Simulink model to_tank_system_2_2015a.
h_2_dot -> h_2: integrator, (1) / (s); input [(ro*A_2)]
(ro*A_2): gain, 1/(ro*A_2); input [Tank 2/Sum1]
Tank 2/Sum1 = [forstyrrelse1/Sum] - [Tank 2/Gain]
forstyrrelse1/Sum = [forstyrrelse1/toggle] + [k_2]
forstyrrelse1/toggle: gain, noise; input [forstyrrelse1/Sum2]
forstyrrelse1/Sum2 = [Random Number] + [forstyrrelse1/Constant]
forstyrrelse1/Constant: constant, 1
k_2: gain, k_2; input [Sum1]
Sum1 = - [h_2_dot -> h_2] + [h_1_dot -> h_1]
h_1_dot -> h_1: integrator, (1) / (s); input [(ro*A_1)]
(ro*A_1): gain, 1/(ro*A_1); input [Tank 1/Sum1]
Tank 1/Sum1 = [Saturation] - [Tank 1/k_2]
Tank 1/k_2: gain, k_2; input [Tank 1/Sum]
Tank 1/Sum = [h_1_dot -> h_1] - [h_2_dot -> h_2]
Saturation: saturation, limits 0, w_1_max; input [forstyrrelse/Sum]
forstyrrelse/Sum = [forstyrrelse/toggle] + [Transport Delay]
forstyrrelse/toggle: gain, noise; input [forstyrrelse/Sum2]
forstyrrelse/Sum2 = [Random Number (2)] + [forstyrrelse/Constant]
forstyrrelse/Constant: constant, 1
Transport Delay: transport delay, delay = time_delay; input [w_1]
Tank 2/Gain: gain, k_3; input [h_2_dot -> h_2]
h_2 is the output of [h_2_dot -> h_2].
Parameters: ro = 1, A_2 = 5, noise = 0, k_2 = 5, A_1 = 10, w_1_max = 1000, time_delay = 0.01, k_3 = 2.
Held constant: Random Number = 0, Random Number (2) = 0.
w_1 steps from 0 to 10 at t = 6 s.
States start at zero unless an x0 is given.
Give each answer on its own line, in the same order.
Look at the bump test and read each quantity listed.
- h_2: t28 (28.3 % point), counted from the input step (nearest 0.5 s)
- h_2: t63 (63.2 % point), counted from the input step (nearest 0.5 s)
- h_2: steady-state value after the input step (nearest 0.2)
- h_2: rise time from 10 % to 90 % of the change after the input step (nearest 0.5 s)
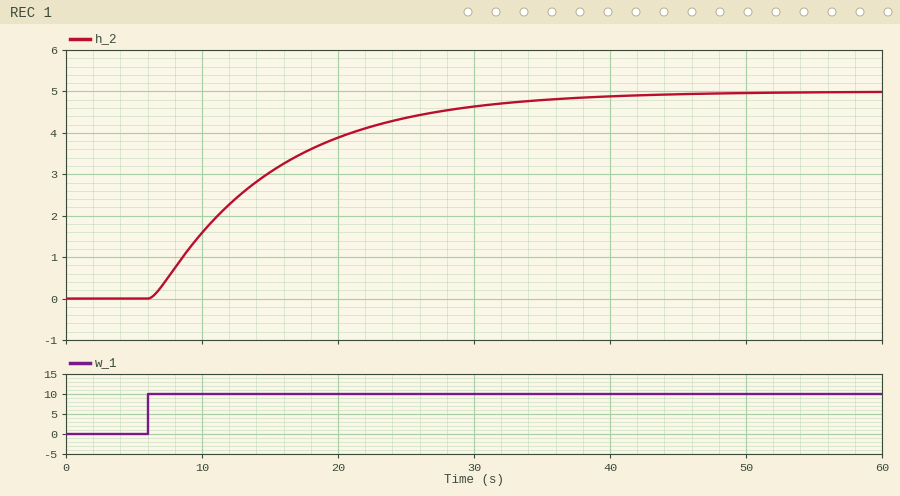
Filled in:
3.5 s
9.5 s
5.0
19.5 s
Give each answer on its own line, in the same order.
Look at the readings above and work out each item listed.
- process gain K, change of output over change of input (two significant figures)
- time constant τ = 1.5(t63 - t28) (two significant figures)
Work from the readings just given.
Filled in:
0.50
9.0 s
